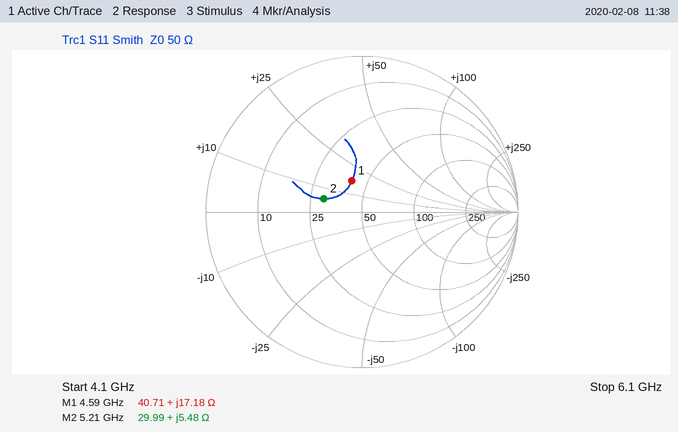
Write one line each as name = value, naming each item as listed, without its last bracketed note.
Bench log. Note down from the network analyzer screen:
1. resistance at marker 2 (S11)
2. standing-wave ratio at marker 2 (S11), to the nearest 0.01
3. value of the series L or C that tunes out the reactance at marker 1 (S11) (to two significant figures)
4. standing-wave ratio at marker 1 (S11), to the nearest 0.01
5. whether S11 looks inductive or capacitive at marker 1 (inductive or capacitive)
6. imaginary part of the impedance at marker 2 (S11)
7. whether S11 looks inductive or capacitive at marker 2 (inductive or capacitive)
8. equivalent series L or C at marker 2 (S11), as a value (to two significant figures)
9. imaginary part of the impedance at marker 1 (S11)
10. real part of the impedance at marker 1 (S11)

resistance at marker 2 = 29.99 Ω
standing-wave ratio at marker 2 (S11), to the nearest 0.01 = 1.70
value of the series L or C that tunes out the reactance at marker 1 (S11) = 2.0 pF
standing-wave ratio at marker 1 (S11), to the nearest 0.01 = 1.54
whether S11 looks inductive or capacitive at marker 1 = inductive
imaginary part of the impedance at marker 2 = +5.48 Ω
whether S11 looks inductive or capacitive at marker 2 = inductive
equivalent series L or C at marker 2 (S11), as a value = 170 pH
imaginary part of the impedance at marker 1 = +17.18 Ω
real part of the impedance at marker 1 = 40.71 Ω
